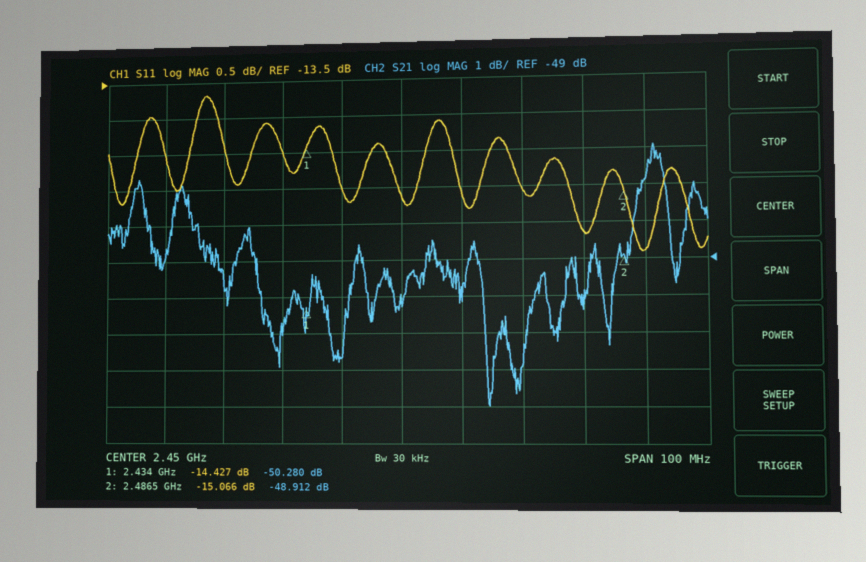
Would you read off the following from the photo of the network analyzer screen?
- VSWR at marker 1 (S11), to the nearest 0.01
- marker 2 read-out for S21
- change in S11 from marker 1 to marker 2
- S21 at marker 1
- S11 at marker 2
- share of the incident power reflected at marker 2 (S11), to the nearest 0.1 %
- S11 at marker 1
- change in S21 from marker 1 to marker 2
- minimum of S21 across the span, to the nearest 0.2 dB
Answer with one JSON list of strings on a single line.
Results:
["1.47", "-48.912 dB", "-0.639 dB", "-50.280 dB", "-15.066 dB", "3.1 %", "-14.427 dB", "1.368 dB", "-53.0 dB"]
